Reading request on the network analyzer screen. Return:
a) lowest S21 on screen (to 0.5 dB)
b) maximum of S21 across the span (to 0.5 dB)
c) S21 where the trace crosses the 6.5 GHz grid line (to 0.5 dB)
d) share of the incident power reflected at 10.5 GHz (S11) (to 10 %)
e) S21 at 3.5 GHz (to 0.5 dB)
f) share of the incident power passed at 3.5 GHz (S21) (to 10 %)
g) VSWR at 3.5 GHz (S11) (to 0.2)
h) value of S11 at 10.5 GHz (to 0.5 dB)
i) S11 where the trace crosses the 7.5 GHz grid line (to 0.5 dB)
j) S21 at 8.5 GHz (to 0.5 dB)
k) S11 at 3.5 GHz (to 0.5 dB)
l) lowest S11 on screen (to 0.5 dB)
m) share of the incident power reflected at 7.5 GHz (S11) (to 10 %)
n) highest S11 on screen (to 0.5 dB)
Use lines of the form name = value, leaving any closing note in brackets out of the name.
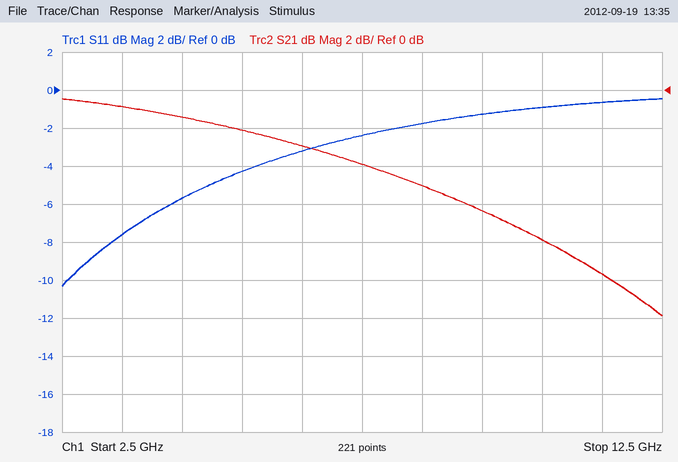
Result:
lowest S21 on screen = -12.0 dB
maximum of S21 across the span = -0.5 dB
S21 where the trace crosses the 6.5 GHz grid line = -3.0 dB
share of the incident power reflected at 10.5 GHz (S11) = 80 %
S21 at 3.5 GHz = -1.0 dB
share of the incident power passed at 3.5 GHz (S21) = 80 %
VSWR at 3.5 GHz (S11) = 2.4
value of S11 at 10.5 GHz = -1.0 dB
S11 where the trace crosses the 7.5 GHz grid line = -2.5 dB
S21 at 8.5 GHz = -5.0 dB
S11 at 3.5 GHz = -7.5 dB
lowest S11 on screen = -10.5 dB
share of the incident power reflected at 7.5 GHz (S11) = 60 %
highest S11 on screen = -0.5 dB
